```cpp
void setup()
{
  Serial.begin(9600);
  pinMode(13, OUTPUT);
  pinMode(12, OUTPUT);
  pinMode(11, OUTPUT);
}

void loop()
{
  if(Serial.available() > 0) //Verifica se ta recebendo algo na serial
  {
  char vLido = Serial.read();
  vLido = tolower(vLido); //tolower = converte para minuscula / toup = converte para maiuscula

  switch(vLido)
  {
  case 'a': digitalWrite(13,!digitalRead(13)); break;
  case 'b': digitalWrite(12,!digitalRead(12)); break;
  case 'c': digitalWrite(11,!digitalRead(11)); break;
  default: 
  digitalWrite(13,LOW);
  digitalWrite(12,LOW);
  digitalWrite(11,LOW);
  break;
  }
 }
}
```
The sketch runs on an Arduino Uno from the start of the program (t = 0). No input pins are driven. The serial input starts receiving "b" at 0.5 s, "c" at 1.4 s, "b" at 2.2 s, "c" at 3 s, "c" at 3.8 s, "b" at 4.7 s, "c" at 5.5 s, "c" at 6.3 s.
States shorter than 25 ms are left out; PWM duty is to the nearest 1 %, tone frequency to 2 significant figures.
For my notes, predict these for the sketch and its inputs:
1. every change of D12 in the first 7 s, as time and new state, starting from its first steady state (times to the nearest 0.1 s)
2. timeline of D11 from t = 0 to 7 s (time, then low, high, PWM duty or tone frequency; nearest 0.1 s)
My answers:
0 s low; 0.5 s high; 2.2 s low; 4.7 s high
0 s low; 1.4 s high; 3 s low; 3.8 s high; 5.5 s low; 6.3 s high
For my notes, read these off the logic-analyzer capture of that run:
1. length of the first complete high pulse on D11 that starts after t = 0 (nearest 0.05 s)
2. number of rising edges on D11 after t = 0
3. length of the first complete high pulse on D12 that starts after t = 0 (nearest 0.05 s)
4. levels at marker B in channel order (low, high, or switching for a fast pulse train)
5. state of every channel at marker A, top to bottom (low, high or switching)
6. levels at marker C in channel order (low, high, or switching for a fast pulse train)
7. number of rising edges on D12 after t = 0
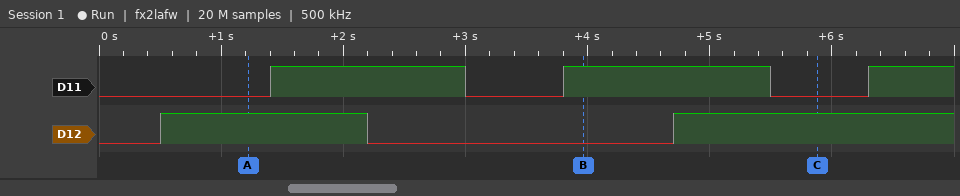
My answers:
1.60 s
3
1.70 s
D11 high, D12 low
D11 low, D12 high
D11 low, D12 high
2
